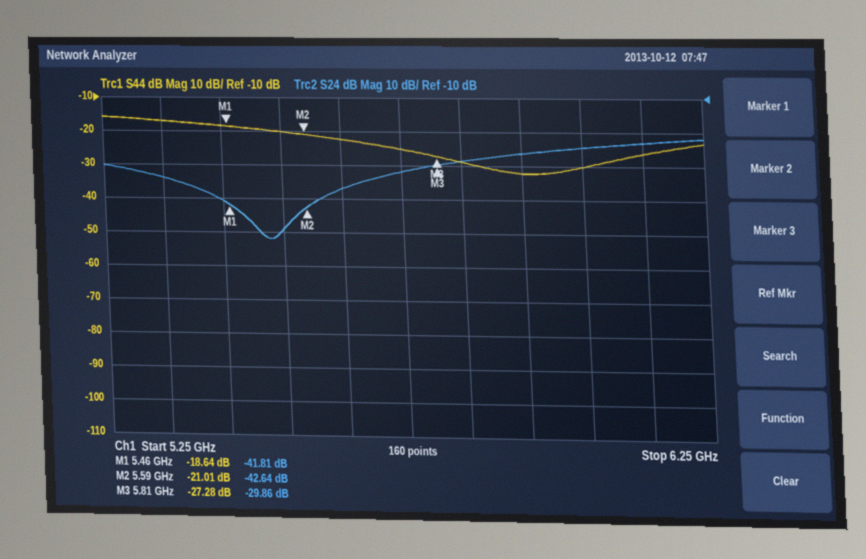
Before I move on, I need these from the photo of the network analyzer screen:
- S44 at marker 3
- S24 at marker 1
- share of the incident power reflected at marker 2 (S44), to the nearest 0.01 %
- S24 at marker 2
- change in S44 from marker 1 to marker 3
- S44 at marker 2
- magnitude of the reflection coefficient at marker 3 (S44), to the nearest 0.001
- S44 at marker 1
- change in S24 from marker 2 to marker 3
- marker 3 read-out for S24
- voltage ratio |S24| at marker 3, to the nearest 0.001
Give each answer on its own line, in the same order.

-27.28 dB
-41.81 dB
0.79 %
-42.64 dB
-8.64 dB
-21.01 dB
0.043
-18.64 dB
12.78 dB
-29.86 dB
0.032
